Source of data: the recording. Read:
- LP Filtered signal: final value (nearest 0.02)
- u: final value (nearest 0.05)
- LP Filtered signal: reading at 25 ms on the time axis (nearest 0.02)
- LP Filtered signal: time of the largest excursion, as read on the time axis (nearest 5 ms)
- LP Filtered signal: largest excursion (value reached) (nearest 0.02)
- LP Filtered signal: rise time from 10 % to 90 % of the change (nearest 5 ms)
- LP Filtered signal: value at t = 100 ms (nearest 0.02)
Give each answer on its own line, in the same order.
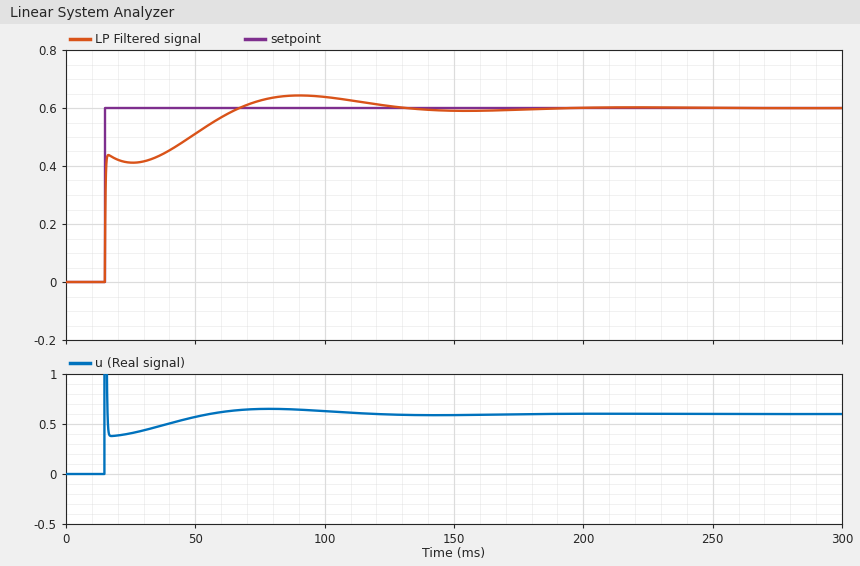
0.60
0.60
0.42
90 ms
0.64
40 ms
0.64
